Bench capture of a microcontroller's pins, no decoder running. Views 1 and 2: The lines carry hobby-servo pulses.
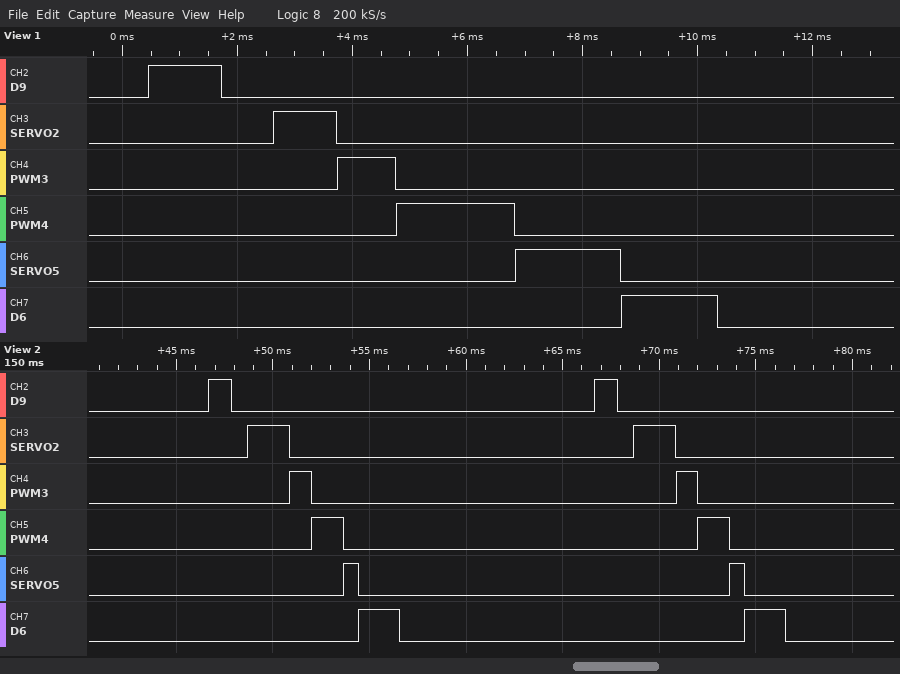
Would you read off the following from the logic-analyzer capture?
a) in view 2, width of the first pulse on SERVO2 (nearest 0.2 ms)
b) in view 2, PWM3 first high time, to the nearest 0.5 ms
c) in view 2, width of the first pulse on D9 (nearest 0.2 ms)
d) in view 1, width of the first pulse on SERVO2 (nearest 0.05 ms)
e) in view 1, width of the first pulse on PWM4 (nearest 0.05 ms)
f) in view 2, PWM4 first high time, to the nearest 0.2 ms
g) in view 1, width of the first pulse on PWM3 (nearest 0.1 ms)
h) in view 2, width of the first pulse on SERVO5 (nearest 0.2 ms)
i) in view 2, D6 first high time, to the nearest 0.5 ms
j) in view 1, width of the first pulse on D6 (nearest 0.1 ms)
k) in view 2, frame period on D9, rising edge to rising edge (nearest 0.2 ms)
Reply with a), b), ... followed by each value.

a) 2.2 ms
b) 1.0 ms
c) 1.2 ms
d) 1.10 ms
e) 2.05 ms
f) 1.6 ms
g) 1.0 ms
h) 0.8 ms
i) 2.0 ms
j) 1.7 ms
k) 20.0 ms
